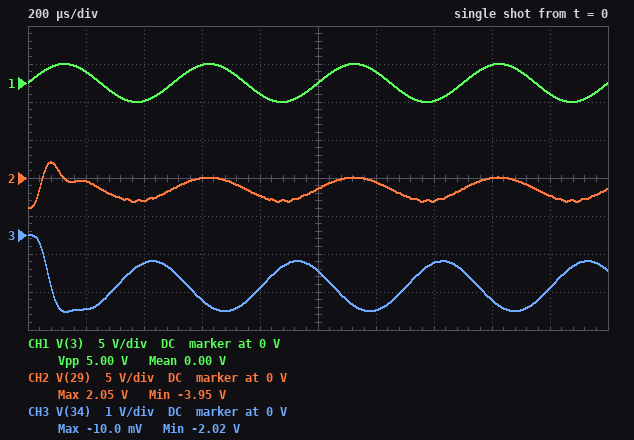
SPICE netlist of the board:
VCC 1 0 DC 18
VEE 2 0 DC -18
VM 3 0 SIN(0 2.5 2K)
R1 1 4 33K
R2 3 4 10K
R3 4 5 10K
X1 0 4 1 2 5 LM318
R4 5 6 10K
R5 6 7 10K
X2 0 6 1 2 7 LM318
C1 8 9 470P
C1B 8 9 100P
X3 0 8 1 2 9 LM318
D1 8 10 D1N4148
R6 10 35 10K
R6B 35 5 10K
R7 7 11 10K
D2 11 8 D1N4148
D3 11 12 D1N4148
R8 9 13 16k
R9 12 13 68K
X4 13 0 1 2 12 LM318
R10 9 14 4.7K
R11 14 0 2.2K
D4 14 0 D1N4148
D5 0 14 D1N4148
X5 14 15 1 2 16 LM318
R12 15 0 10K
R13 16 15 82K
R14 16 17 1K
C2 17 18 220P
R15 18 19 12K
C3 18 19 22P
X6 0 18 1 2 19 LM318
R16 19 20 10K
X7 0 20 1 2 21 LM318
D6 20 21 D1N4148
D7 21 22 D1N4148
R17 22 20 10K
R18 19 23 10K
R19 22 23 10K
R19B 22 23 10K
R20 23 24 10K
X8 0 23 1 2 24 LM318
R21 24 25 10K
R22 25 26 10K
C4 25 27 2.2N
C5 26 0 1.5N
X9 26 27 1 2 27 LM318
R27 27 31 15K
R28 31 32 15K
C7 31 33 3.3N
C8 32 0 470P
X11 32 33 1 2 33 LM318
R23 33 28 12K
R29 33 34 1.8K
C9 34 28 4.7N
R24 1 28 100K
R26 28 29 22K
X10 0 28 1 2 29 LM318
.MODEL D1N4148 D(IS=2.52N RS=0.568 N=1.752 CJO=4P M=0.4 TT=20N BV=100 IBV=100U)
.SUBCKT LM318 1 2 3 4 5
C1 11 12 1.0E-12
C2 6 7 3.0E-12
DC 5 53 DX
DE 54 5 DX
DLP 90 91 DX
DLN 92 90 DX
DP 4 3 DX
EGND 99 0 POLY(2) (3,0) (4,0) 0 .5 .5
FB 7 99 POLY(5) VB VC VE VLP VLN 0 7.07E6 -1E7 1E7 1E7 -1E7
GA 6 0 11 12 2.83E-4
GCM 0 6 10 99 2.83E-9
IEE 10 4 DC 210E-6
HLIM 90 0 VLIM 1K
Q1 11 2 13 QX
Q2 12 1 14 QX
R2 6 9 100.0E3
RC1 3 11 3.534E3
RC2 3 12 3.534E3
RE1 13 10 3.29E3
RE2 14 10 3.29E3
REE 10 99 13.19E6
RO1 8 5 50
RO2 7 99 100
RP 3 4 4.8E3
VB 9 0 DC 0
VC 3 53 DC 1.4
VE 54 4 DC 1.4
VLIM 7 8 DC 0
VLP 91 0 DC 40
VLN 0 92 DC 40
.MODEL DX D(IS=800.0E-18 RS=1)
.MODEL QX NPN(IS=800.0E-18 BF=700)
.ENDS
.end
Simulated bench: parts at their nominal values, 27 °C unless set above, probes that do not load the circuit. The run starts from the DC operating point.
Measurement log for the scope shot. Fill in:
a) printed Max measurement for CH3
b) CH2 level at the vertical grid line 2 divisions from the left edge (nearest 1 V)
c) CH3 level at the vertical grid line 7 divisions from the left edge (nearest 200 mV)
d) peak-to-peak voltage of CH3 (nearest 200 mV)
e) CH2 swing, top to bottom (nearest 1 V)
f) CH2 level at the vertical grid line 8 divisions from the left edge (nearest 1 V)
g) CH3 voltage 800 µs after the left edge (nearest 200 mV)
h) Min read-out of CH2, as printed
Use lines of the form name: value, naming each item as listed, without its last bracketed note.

printed Max measurement for CH3: -10.0 mV
CH2 level at the vertical grid line 2 divisions from the left edge: -3 V
CH3 level at the vertical grid line 7 divisions from the left edge: -800 mV
peak-to-peak voltage of CH3: 2.0 V
CH2 swing, top to bottom: 6 V
CH2 level at the vertical grid line 8 divisions from the left edge: 0 V
CH3 voltage 800 µs after the left edge: -1.4 V
Min read-out of CH2, as printed: -3.95 V
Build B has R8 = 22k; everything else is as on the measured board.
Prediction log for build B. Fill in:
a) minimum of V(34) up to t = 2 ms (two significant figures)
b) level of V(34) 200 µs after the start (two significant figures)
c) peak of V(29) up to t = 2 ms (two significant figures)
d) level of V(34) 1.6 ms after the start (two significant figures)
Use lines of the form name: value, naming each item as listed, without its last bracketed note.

minimum of V(34) up to t = 2 ms: -1.6 V
level of V(34) 200 µs after the start: -1.5 V
peak of V(29) up to t = 2 ms: 600 mV
level of V(34) 1.6 ms after the start: -1.3 V
